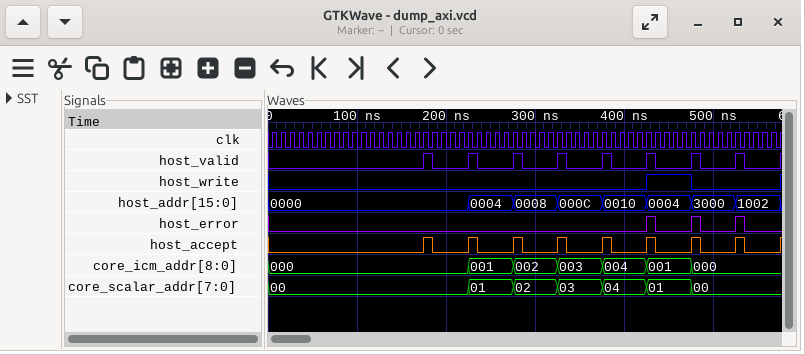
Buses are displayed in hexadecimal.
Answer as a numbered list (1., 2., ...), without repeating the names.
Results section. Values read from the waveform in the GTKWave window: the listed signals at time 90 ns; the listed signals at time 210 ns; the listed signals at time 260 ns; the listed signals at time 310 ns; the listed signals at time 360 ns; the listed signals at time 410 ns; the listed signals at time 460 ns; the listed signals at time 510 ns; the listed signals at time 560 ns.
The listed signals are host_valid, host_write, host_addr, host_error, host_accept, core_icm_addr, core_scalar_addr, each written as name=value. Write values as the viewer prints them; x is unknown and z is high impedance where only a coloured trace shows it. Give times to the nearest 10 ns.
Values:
1. host_valid=0, host_write=0, host_addr=0000, host_error=0, host_accept=0, core_icm_addr=000, core_scalar_addr=00
2. host_valid=0, host_write=0, host_addr=0000, host_error=0, host_accept=0, core_icm_addr=000, core_scalar_addr=00
3. host_valid=0, host_write=0, host_addr=0004, host_error=0, host_accept=0, core_icm_addr=001, core_scalar_addr=01
4. host_valid=0, host_write=0, host_addr=0008, host_error=0, host_accept=0, core_icm_addr=002, core_scalar_addr=02
5. host_valid=0, host_write=0, host_addr=000C, host_error=0, host_accept=0, core_icm_addr=003, core_scalar_addr=03
6. host_valid=0, host_write=0, host_addr=0010, host_error=0, host_accept=0, core_icm_addr=004, core_scalar_addr=04
7. host_valid=0, host_write=1, host_addr=0004, host_error=0, host_accept=0, core_icm_addr=001, core_scalar_addr=01
8. host_valid=0, host_write=0, host_addr=3000, host_error=0, host_accept=0, core_icm_addr=000, core_scalar_addr=00
9. host_valid=0, host_write=0, host_addr=1002, host_error=0, host_accept=0, core_icm_addr=000, core_scalar_addr=00
